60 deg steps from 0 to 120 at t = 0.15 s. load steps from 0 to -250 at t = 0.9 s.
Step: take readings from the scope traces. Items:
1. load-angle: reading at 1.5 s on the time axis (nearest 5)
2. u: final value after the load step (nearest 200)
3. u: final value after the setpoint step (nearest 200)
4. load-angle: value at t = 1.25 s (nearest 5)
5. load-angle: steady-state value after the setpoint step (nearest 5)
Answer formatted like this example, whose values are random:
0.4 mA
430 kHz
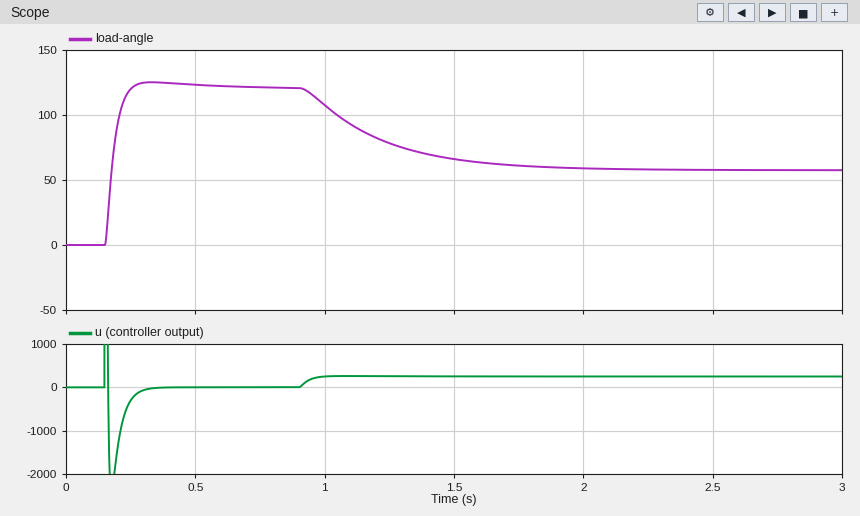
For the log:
65
200
0
80
120
